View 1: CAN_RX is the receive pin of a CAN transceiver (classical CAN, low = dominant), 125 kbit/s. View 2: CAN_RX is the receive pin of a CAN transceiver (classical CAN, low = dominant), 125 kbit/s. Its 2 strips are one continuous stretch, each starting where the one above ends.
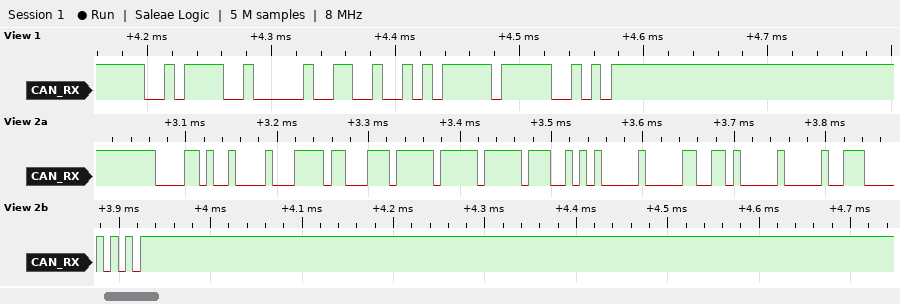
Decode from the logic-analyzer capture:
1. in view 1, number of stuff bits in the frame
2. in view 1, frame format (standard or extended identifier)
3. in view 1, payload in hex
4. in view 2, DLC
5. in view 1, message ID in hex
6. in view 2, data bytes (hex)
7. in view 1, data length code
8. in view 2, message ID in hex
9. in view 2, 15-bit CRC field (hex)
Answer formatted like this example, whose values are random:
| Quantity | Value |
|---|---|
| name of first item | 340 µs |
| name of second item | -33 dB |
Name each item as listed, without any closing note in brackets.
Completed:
| Quantity | Value |
|---|---|
| in view 1, number of stuff bits in the frame | 3 |
| in view 1, frame format | standard |
| in view 1, payload in hex | 92 |
| in view 2, DLC | 8 |
| in view 1, message ID in hex | 0x2F2 |
| in view 2, data bytes | F6 3B FF FF 2A 00 4D 00 |
| in view 1, data length code | 1 |
| in view 2, message ID in hex | 0x0D2 |
| in view 2, 15-bit CRC field | 0x070A |
